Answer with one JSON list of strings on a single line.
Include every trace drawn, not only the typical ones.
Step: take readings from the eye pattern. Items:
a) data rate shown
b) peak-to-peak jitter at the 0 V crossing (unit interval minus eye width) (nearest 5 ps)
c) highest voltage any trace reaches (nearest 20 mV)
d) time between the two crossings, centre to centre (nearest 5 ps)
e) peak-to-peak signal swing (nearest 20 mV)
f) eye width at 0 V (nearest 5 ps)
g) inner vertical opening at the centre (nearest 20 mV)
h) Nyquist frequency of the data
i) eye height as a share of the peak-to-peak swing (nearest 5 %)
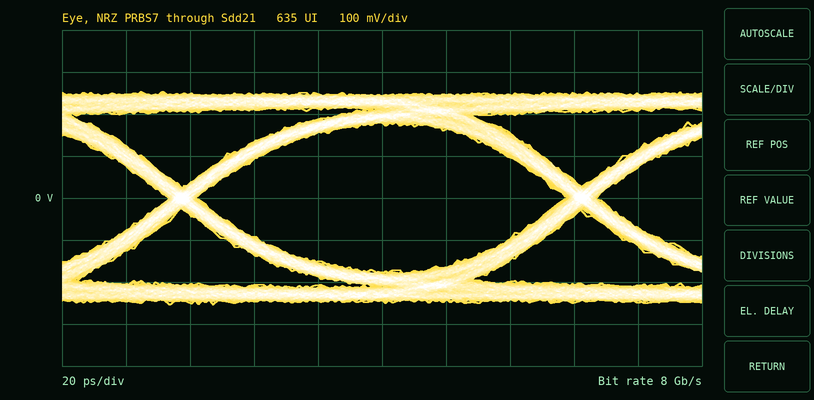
["8 Gb/s", "10 ps", "260 mV", "125 ps", "500 mV", "115 ps", "360 mV", "4 GHz", "70 %"]
